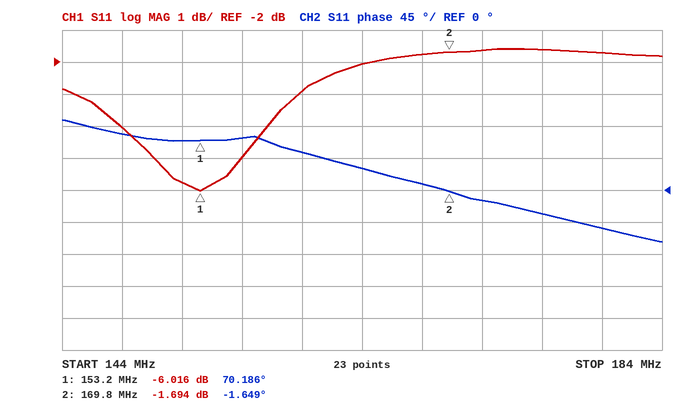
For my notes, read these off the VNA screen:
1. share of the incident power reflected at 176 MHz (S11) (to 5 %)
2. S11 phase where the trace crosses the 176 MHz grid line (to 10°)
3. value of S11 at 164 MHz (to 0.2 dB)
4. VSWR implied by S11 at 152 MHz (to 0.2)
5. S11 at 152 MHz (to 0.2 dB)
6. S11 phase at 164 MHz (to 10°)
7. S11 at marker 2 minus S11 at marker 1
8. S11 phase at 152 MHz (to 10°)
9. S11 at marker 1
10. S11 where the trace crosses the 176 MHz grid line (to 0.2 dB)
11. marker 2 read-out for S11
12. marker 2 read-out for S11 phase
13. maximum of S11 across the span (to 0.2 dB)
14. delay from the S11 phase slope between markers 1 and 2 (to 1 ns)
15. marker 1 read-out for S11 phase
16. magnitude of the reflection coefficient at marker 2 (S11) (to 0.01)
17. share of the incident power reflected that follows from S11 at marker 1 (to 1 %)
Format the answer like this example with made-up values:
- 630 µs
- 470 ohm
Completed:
- 70 %
- -30°
- -2.0 dB
- 3.2
- -5.8 dB
- 30°
- 4.322 dB
- 70°
- -6.016 dB
- -1.6 dB
- -1.694 dB
- -1.649°
- -1.6 dB
- 12 ns
- 70.186°
- 0.82
- 25 %
